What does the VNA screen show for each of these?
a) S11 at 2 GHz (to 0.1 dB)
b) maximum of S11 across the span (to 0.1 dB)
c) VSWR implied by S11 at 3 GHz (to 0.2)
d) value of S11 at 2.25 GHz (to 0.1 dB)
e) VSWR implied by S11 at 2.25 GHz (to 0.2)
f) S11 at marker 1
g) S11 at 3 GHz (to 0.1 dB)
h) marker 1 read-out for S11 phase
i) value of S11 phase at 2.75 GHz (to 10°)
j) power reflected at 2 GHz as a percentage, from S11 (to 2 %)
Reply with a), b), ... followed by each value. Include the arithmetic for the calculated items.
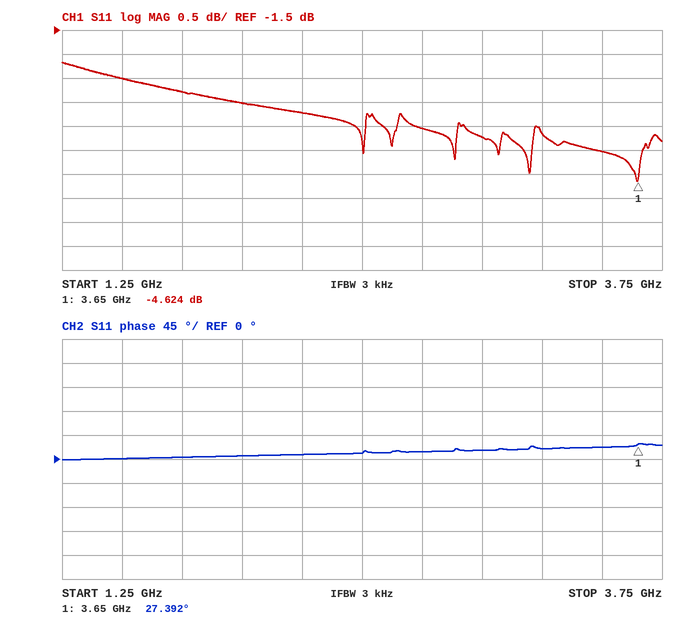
a) -3.0 dB
b) -2.2 dB
c) |Γ| = 10^(-3.7/20) = 0.6531; VSWR = (1 + 0.6531)/(1 − 0.6531) ≈ 4.8
d) -3.2 dB
e) |Γ| = 10^(-3.2/20) = 0.6918; VSWR = (1 + 0.6918)/(1 − 0.6918) ≈ 5.49, so 5.4 to the nearest 0.2
f) -4.624 dB
g) -3.7 dB
h) 27.392°
i) 10°
j) 10^(-3/10) ≈ 50 %
